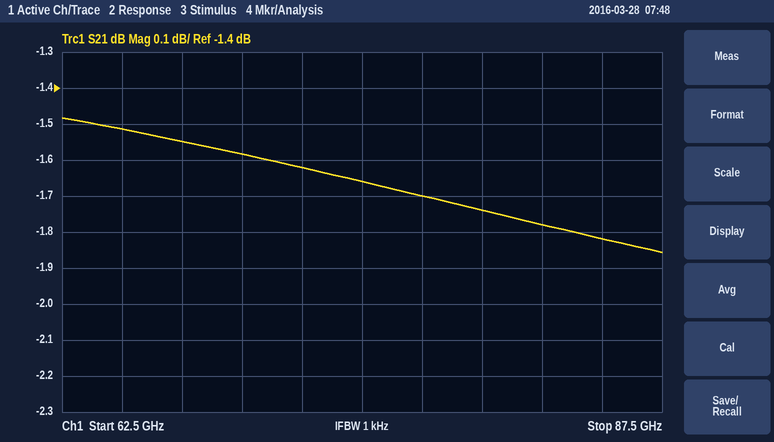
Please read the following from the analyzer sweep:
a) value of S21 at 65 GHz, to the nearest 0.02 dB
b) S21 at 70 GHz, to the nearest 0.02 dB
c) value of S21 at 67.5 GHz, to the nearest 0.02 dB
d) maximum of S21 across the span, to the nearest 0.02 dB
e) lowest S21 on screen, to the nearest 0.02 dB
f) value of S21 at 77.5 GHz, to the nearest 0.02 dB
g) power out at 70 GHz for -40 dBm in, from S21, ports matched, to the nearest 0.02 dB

-1.52 dB
-1.58 dB
-1.54 dB
-1.48 dB
-1.86 dB
-1.70 dB
-41.58 dBm
